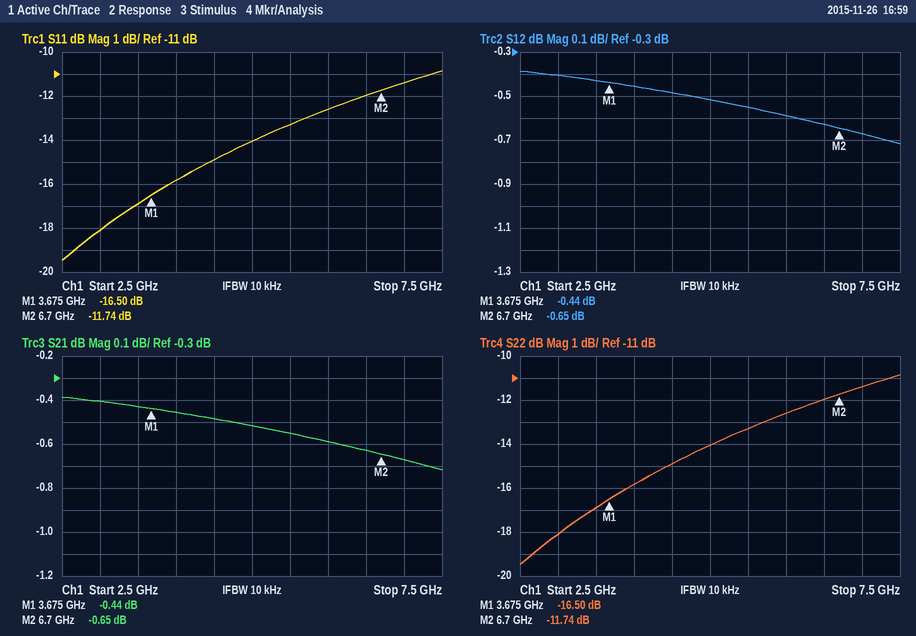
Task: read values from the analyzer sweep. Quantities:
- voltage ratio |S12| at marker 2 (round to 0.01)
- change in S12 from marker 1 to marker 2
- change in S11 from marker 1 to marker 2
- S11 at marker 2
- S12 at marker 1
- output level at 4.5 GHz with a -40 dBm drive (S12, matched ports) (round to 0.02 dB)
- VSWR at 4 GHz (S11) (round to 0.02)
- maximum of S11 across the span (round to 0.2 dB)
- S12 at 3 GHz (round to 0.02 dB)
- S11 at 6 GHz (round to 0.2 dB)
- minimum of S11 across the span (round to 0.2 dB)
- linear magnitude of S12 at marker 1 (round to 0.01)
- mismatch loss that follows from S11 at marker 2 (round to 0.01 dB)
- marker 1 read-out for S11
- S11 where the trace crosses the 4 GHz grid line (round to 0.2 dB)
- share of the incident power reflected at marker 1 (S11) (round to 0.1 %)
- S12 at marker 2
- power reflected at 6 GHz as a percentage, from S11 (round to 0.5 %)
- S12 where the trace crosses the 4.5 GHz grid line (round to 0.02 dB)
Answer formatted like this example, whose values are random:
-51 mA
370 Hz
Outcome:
0.93
-0.21 dB
4.76 dB
-11.74 dB
-0.44 dB
-40.48 dBm
1.38
-10.8 dB
-0.40 dB
-12.6 dB
-19.4 dB
0.95
0.30 dB
-16.50 dB
-15.8 dB
2.2 %
-0.65 dB
5.5 %
-0.48 dB
